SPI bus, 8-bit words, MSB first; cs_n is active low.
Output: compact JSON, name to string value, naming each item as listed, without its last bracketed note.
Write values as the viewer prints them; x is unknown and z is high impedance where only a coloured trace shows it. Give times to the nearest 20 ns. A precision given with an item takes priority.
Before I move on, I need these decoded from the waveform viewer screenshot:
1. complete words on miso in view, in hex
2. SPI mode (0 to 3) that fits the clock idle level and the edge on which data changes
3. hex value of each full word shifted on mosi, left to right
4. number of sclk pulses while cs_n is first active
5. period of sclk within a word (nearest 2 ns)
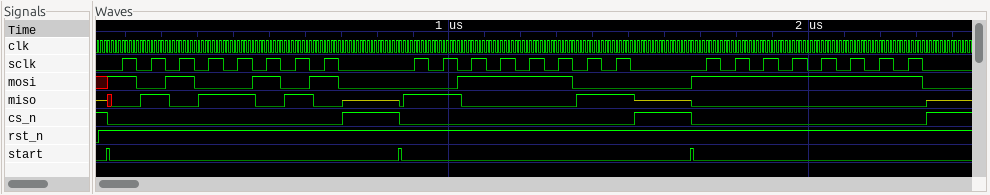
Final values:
{"complete words on miso in view, in hex": "5A, C3, 00", "SPI mode (0 to 3) that fits the clock idle level and the edge on which data changes": "0", "hex value of each full word shifted on mosi, left to right": "A5, 3C, FF", "number of sclk pulses while cs_n is first active": "8", "period of sclk within a word": "80 ns"}
